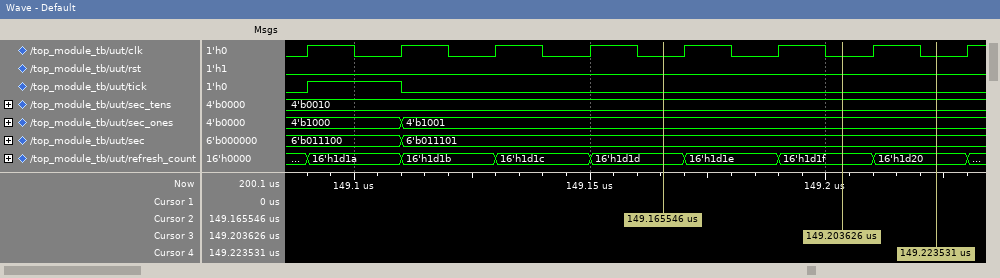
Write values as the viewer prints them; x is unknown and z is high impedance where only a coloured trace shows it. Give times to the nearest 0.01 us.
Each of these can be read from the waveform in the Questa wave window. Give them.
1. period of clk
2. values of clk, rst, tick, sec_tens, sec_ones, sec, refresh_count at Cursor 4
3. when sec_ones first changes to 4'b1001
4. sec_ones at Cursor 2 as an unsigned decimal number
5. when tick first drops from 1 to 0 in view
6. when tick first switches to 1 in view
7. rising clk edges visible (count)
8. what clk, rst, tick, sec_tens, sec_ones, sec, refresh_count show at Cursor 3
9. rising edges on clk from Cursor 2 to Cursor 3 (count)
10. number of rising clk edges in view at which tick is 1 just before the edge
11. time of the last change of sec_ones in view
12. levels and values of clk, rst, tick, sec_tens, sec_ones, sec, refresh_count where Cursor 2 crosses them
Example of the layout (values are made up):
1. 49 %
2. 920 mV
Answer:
1. 0.02 us
2. clk=0, rst=0, tick=0, sec_tens=4'b0010, sec_ones=4'b1001, sec=6'b011101, refresh_count=16'h1d20
3. 149.11 us
4. 9
5. 149.11 us
6. 149.09 us
7. 8
8. clk=0, rst=0, tick=0, sec_tens=4'b0010, sec_ones=4'b1001, sec=6'b011101, refresh_count=16'h1d1f
9. 2
10. 1
11. 149.11 us
12. clk=0, rst=0, tick=0, sec_tens=4'b0010, sec_ones=4'b1001, sec=6'b011101, refresh_count=16'h1d1d
